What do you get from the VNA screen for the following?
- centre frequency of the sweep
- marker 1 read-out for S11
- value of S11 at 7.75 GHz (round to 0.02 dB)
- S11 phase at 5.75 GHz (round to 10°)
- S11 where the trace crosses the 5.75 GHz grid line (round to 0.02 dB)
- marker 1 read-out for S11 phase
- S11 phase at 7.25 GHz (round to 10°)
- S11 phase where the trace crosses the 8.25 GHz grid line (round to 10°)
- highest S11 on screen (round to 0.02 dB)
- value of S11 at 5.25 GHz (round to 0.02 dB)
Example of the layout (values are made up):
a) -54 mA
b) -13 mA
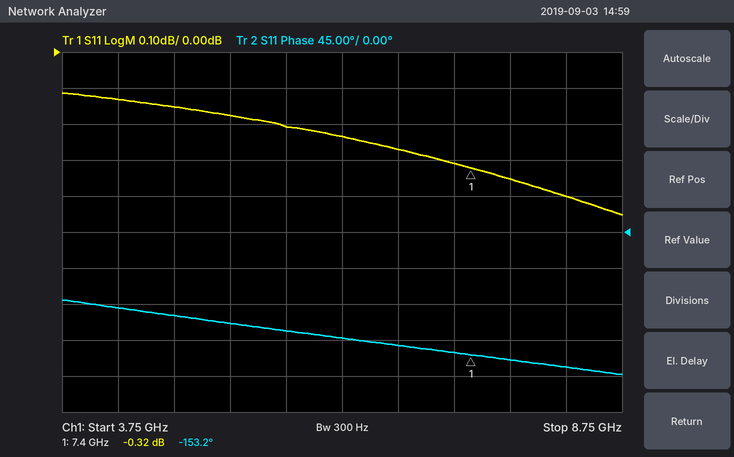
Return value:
a) 6.25 GHz
b) -0.32 dB
c) -0.36 dB
d) -120°
e) -0.20 dB
f) -153.2°
g) -150°
h) -170°
i) -0.12 dB
j) -0.18 dB
